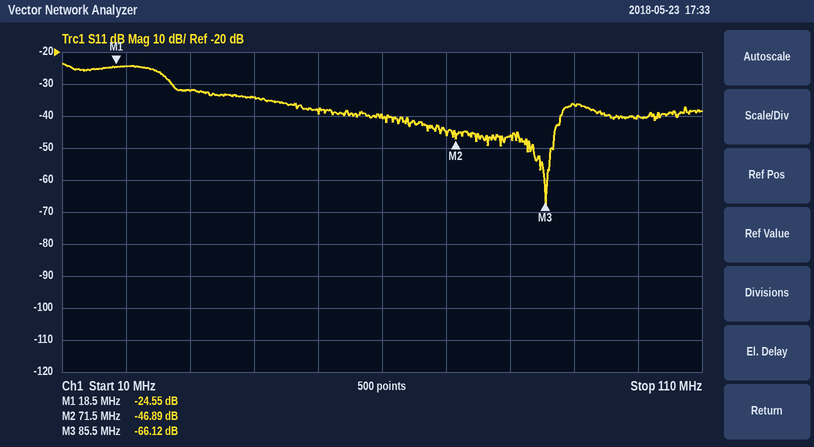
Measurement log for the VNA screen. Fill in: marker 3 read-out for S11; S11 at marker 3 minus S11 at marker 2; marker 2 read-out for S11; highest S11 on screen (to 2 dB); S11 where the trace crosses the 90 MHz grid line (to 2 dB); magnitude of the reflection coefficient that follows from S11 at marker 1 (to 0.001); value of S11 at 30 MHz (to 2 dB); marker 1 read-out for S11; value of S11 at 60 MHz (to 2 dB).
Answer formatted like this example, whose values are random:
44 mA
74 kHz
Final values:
-66.12 dB
-19.23 dB
-46.89 dB
-24 dB
-36 dB
0.059
-32 dB
-24.55 dB
-40 dB
